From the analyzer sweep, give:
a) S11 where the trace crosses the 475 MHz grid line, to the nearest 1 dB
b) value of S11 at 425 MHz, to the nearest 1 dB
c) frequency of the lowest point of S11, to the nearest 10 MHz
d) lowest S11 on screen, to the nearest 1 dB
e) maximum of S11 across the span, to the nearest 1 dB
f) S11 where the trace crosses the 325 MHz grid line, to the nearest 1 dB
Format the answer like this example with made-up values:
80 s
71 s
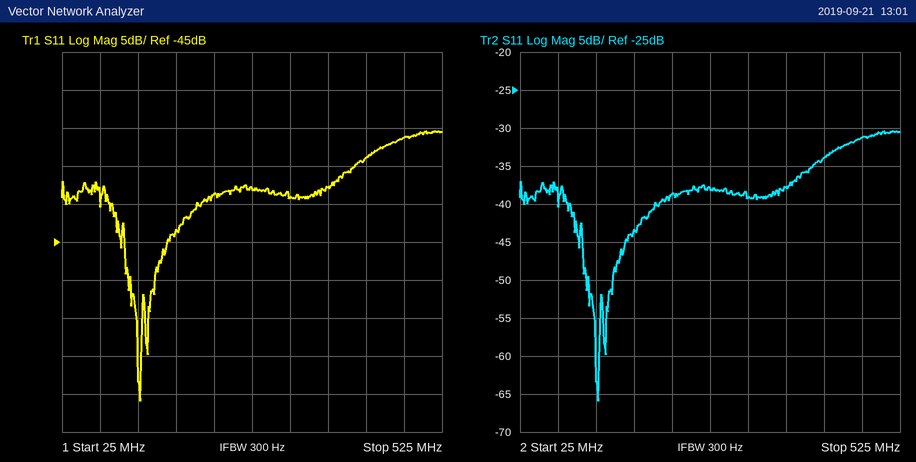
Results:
-31 dB
-34 dB
130 MHz
-66 dB
-30 dB
-39 dB
